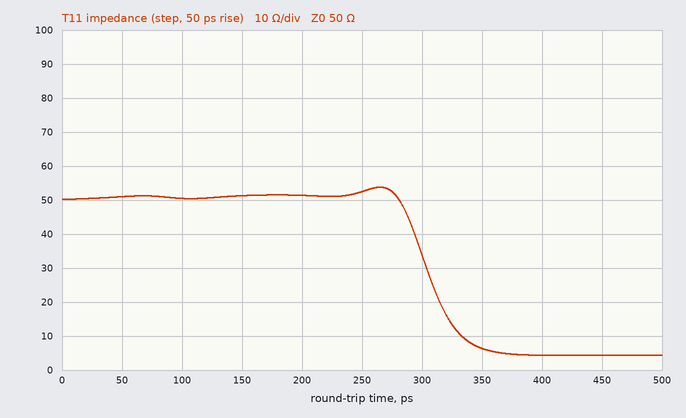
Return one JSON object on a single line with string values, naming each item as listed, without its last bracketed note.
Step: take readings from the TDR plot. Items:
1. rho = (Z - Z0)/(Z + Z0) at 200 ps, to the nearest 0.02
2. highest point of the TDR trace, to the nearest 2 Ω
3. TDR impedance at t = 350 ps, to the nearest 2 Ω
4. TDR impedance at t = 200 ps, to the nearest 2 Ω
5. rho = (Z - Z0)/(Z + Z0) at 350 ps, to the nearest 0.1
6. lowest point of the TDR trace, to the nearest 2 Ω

{"rho = (Z - Z0)/(Z + Z0) at 200 ps, to the nearest 0.02": "+0.02", "highest point of the TDR trace, to the nearest 2 Ω": "54 Ω", "TDR impedance at t = 350 ps, to the nearest 2 Ω": "6 Ω", "TDR impedance at t = 200 ps, to the nearest 2 Ω": "52 Ω", "rho = (Z - Z0)/(Z + Z0) at 350 ps, to the nearest 0.1": "-0.8", "lowest point of the TDR trace, to the nearest 2 Ω": "4 Ω"}
